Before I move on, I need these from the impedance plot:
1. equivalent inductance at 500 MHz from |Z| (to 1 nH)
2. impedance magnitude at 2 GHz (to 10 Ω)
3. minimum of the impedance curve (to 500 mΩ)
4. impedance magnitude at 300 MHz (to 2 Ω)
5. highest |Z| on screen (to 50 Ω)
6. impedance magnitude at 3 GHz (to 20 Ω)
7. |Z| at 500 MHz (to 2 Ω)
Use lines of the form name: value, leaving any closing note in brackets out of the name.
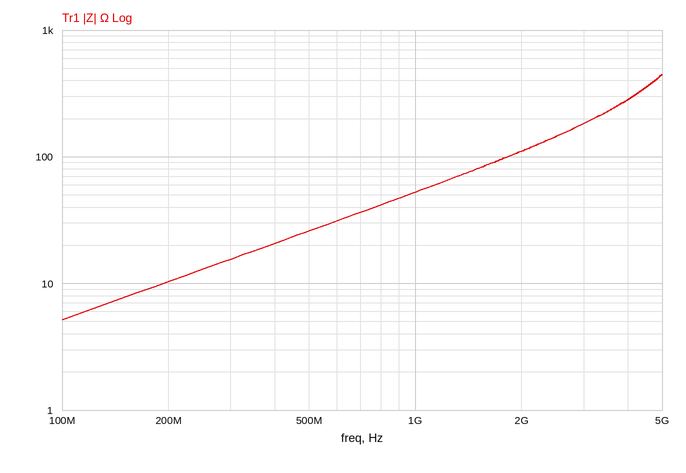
equivalent inductance at 500 MHz from |Z|: 8 nH
impedance magnitude at 2 GHz: 110 Ω
minimum of the impedance curve: 5.0 Ω
impedance magnitude at 300 MHz: 16 Ω
highest |Z| on screen: 450 Ω
impedance magnitude at 3 GHz: 180 Ω
|Z| at 500 MHz: 26 Ω
